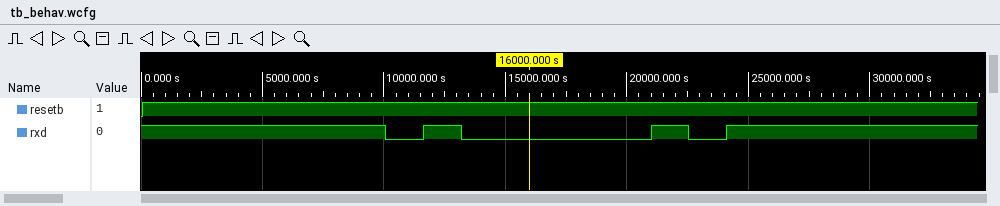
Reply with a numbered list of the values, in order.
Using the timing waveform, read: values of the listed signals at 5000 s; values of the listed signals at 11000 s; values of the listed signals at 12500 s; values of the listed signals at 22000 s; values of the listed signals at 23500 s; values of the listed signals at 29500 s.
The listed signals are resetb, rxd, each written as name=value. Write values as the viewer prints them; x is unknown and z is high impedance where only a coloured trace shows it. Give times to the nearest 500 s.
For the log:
1. resetb=1, rxd=1
2. resetb=1, rxd=0
3. resetb=1, rxd=1
4. resetb=1, rxd=1
5. resetb=1, rxd=0
6. resetb=1, rxd=1
